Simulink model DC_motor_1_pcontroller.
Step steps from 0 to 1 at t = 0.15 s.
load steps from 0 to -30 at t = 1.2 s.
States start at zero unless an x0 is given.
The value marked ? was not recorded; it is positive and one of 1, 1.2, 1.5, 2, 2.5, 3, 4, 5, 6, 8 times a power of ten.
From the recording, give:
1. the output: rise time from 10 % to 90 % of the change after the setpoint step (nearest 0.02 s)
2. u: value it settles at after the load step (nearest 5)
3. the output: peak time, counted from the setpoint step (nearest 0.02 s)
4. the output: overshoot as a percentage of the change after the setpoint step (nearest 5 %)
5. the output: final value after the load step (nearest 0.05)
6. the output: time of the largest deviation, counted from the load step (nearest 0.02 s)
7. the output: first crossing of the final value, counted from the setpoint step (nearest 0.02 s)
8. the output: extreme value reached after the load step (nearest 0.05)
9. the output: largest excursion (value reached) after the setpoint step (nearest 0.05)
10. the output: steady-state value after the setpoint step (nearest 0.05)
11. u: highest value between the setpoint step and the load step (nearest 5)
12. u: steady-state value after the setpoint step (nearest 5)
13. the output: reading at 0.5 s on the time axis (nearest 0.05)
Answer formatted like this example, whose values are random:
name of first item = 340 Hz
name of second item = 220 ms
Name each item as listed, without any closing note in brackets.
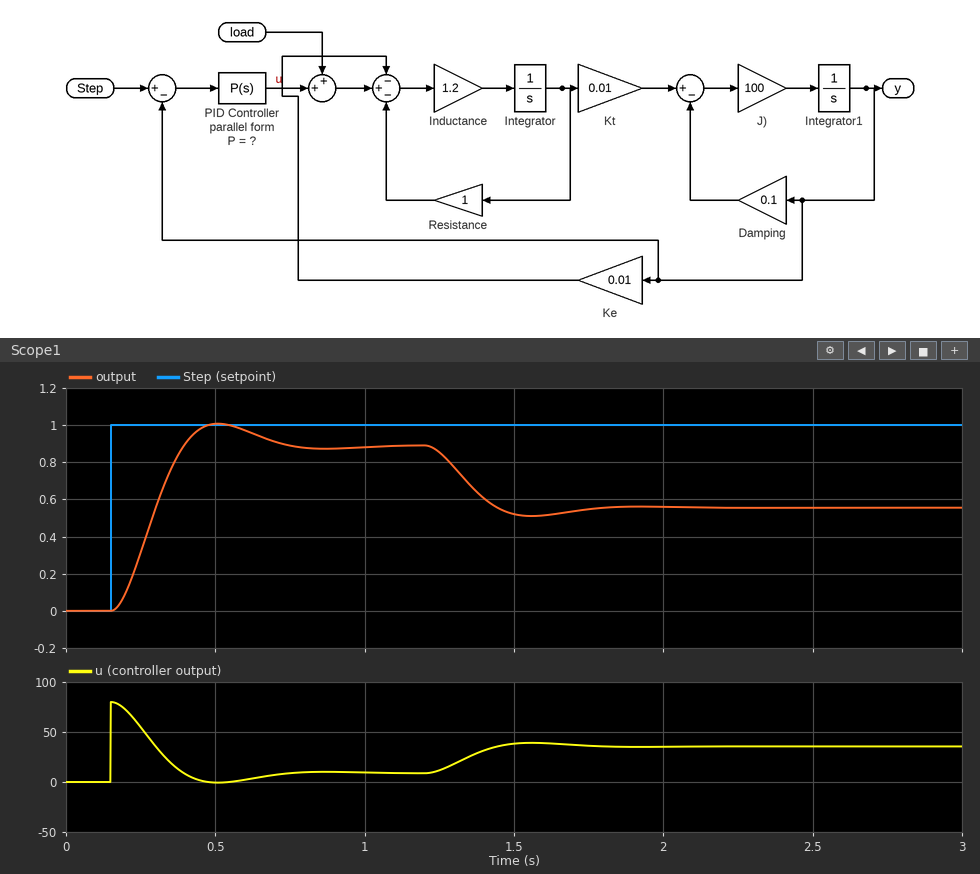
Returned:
the output: rise time from 10 % to 90 % of the change after the setpoint step = 0.16 s
u: value it settles at after the load step = 35
the output: peak time, counted from the setpoint step = 0.36 s
the output: overshoot as a percentage of the change after the setpoint step = 15 %
the output: final value after the load step = 0.55
the output: time of the largest deviation, counted from the load step = 0.36 s
the output: first crossing of the final value, counted from the setpoint step = 0.24 s
the output: extreme value reached after the load step = 0.50
the output: largest excursion (value reached) after the setpoint step = 1.00
the output: steady-state value after the setpoint step = 0.90
u: highest value between the setpoint step and the load step = 80
u: steady-state value after the setpoint step = 10
the output: reading at 0.5 s on the time axis = 1.00
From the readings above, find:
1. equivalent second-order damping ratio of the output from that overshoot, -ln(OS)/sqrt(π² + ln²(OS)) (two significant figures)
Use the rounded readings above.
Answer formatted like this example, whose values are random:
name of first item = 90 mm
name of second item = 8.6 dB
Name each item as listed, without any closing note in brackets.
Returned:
equivalent second-order damping ratio of the output from that overshoot, -ln(OS)/sqrt(π² + ln²(OS)) = 0.52
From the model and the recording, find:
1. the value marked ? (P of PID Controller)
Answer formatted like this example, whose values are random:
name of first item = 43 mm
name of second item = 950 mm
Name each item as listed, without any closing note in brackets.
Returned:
the value marked ? = 80
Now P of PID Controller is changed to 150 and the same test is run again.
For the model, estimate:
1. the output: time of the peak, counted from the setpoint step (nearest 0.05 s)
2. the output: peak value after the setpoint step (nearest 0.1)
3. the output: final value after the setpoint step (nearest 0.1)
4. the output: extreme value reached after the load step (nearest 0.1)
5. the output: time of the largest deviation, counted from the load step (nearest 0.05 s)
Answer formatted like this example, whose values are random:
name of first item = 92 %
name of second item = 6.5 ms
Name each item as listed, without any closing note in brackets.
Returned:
the output: time of the peak, counted from the setpoint step = 0.25 s
the output: peak value after the setpoint step = 1.2
the output: final value after the setpoint step = 0.9
the output: extreme value reached after the load step = 0.7
the output: time of the largest deviation, counted from the load step = 0.25 s
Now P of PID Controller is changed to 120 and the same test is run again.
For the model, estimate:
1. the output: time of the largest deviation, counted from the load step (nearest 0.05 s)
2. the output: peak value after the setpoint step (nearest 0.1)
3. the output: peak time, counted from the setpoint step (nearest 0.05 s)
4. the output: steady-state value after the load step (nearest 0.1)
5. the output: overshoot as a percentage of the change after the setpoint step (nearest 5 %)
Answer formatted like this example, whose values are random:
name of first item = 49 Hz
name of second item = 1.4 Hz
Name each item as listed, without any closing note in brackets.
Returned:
the output: time of the largest deviation, counted from the load step = 0.30 s
the output: peak value after the setpoint step = 1.1
the output: peak time, counted from the setpoint step = 0.30 s
the output: steady-state value after the load step = 0.7
the output: overshoot as a percentage of the change after the setpoint step = 20 %
